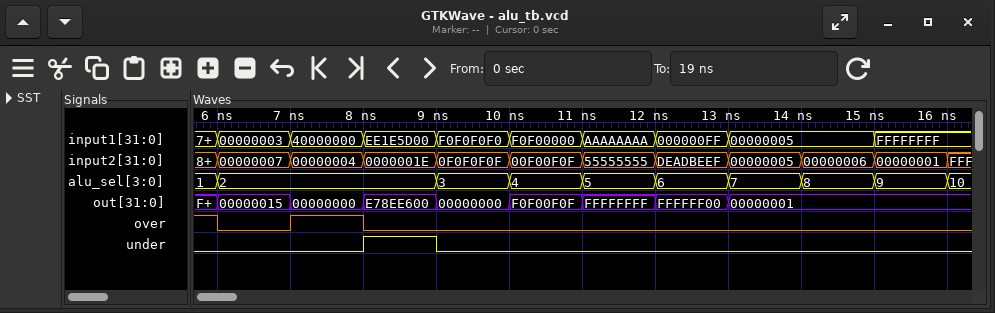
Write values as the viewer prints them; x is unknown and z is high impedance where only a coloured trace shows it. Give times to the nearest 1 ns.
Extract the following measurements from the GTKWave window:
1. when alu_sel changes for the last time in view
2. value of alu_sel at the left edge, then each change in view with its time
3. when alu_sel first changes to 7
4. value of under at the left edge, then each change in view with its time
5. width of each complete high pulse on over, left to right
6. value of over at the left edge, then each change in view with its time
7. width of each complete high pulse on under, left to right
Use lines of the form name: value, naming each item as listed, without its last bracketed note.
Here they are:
when alu_sel changes for the last time in view: 16 ns
value of alu_sel at the left edge, then each change in view with its time: 1, 2 at 6 ns, 3 at 9 ns, 4 at 10 ns, 5 at 11 ns, 6 at 12 ns, 7 at 13 ns, 8 at 14 ns, 9 at 15 ns, 10 at 16 ns
when alu_sel first changes to 7: 13 ns
value of under at the left edge, then each change in view with its time: 0, 1 at 8 ns, 0 at 9 ns
width of each complete high pulse on over, left to right: 1 ns
value of over at the left edge, then each change in view with its time: 1, 0 at 6 ns, 1 at 7 ns, 0 at 8 ns
width of each complete high pulse on under, left to right: 1 ns
